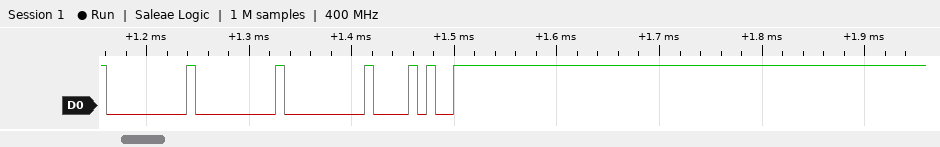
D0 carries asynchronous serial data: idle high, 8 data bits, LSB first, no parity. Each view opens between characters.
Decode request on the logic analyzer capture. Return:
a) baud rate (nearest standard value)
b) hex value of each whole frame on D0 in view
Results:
115200 baud
00, 00, 00, 28
